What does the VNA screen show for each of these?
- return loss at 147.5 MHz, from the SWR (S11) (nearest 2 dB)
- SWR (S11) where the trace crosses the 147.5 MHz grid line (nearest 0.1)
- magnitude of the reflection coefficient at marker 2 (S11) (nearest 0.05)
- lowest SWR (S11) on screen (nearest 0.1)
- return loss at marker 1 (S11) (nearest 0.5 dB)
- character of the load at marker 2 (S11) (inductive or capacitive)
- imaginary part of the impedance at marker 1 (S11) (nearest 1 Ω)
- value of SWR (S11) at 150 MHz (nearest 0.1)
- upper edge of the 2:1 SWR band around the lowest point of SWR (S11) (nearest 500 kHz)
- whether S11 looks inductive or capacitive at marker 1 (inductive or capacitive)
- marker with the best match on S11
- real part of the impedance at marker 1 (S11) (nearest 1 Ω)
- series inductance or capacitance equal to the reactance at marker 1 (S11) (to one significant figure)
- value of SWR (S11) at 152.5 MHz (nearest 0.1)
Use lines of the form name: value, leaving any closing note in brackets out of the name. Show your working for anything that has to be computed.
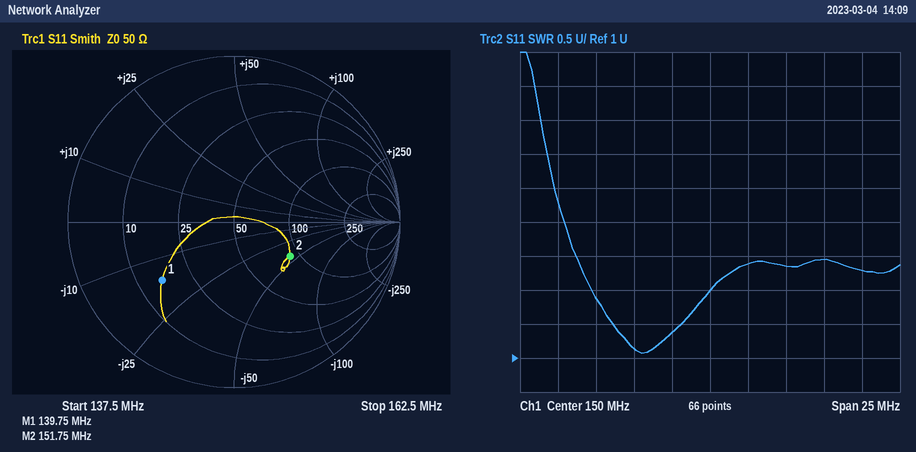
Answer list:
return loss at 147.5 MHz, from the SWR (S11): −20 log10((1.4 − 1)/(1.4 + 1)) ≈ 16 dB
SWR (S11) where the trace crosses the 147.5 MHz grid line: 1.4
magnitude of the reflection coefficient at marker 2 (S11): 0.40
lowest SWR (S11) on screen: 1.1
return loss at marker 1 (S11): 5.0 dB
character of the load at marker 2 (S11): capacitive
imaginary part of the impedance at marker 1 (S11): -16 Ω
value of SWR (S11) at 150 MHz: 2.0
upper edge of the 2:1 SWR band around the lowest point of SWR (S11): 150.0 MHz
whether S11 looks inductive or capacitive at marker 1: capacitive
marker with the best match on S11: marker 2
real part of the impedance at marker 1 (S11): 16 Ω
series inductance or capacitance equal to the reactance at marker 1 (S11): C = 1/(2π × 139.75 MHz × 16 Ω) ≈ 71.2 pF, so 70 pF to one significant figure
value of SWR (S11) at 152.5 MHz: 2.4
